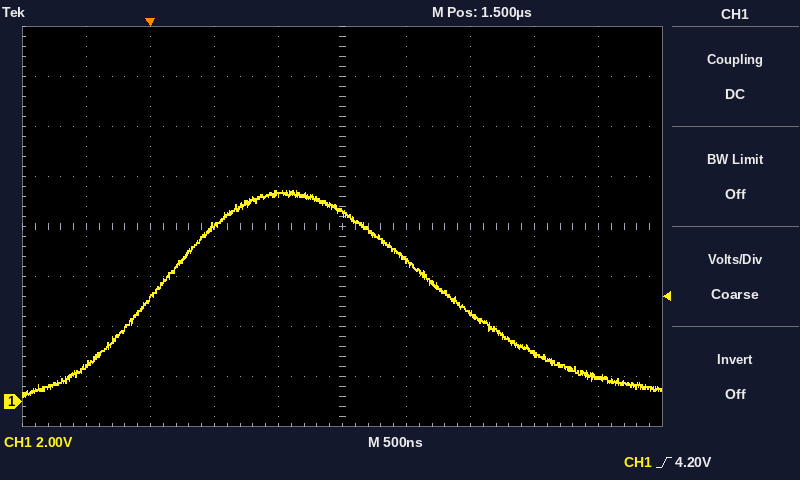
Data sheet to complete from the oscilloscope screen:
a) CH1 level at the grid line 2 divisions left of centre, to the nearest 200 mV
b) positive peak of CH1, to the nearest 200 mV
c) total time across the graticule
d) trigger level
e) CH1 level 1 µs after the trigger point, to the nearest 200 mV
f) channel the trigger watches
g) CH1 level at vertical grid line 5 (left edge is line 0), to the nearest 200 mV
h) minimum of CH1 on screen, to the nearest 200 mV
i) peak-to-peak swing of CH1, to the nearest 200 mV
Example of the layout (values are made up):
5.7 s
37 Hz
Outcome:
7.0 V
8.4 V
5 µs
4.20 V
8.4 V
CH1
7.6 V
200 mV
8.2 V
